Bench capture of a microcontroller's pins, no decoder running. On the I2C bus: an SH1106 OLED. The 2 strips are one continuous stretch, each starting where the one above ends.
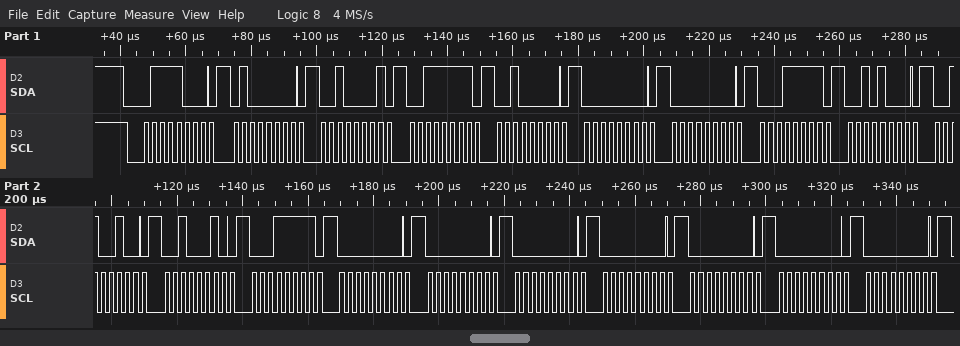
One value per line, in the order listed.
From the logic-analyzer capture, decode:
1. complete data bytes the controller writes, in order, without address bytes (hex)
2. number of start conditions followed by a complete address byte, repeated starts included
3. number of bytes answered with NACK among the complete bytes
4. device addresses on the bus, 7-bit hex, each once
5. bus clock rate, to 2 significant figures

40 21 3F 20 00 00 1F 28 24 22 1F 00 00 00 00 00 00 00
1
0
0x3C
400 kHz
